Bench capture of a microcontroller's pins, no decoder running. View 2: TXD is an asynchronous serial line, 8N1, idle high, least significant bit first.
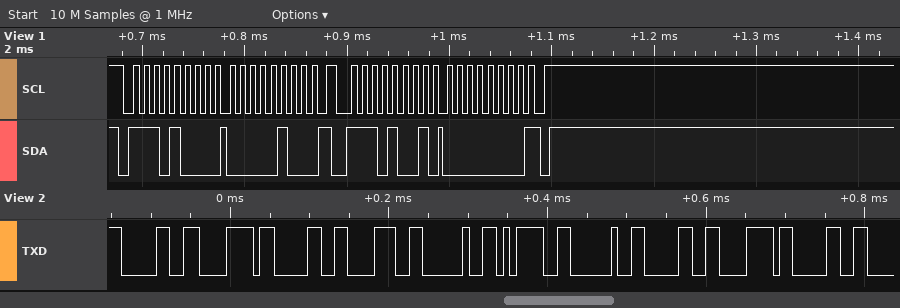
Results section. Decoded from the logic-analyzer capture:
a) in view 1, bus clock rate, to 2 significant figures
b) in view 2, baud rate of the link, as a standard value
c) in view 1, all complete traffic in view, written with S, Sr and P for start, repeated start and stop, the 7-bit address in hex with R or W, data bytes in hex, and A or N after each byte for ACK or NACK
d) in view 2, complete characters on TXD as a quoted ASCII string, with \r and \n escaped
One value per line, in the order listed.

100 kHz
115200 baud
S 74W A 04 A Sr 74R A 00 N P
"0x08 = 0x0"
